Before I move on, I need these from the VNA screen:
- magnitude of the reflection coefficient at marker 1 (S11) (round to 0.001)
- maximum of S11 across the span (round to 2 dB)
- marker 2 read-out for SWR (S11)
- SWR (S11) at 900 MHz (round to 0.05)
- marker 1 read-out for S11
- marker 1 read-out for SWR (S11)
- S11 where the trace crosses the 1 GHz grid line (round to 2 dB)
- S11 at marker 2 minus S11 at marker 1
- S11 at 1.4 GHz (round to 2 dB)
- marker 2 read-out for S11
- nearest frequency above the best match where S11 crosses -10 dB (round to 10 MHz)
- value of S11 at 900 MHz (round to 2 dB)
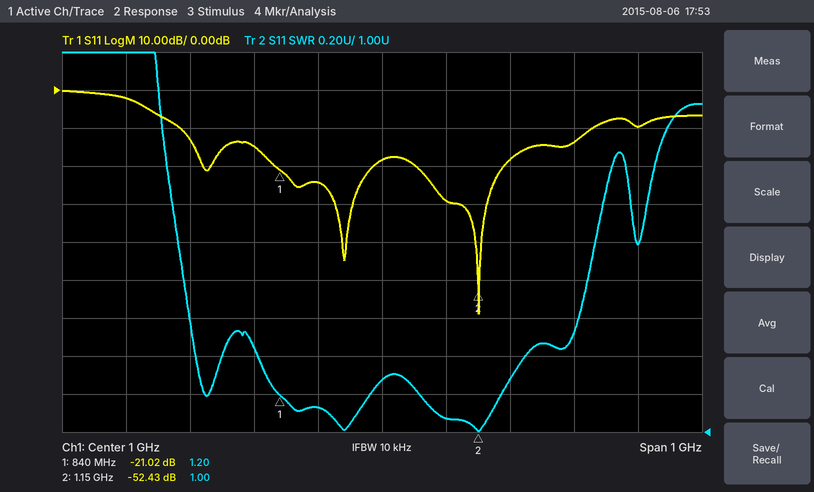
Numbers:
0.089
0 dB
1.00
1.15
-21.02 dB
1.20
-18 dB
-31.41 dB
-10 dB
-52.43 dB
1.33 GHz
-24 dB
